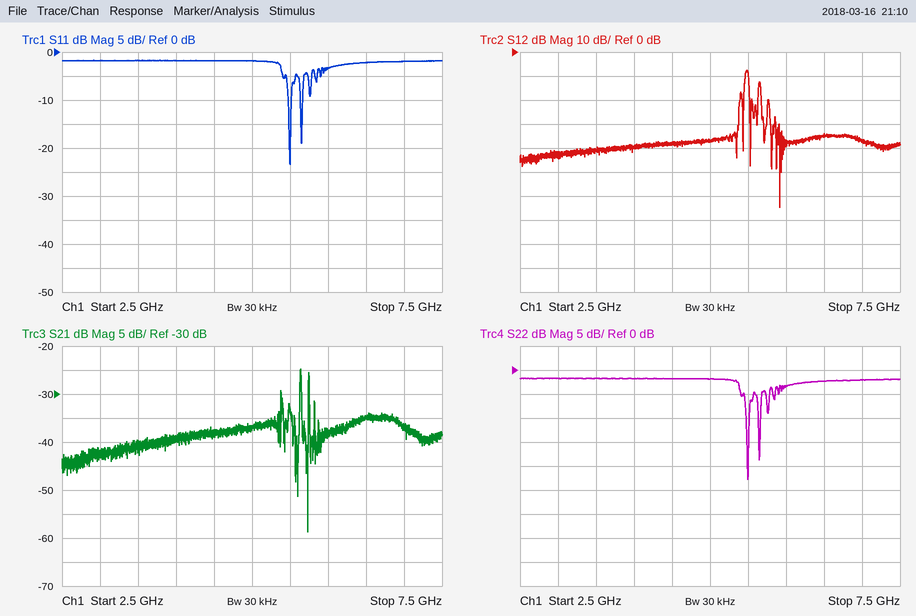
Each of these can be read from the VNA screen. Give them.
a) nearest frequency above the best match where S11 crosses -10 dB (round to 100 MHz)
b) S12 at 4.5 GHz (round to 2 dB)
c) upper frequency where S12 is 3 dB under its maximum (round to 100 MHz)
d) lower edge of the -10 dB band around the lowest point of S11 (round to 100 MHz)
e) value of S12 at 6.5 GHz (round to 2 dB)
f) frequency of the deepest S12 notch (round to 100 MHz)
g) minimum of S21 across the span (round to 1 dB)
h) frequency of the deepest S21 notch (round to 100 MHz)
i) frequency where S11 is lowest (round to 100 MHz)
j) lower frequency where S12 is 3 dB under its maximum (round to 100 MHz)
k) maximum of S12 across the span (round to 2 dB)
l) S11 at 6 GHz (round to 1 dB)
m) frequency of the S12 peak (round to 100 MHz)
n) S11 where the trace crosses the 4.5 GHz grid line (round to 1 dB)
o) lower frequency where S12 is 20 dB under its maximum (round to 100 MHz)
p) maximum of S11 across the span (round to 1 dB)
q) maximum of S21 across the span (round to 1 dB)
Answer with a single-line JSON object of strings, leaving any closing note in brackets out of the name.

{"nearest frequency above the best match where S11 crosses -10 dB": "5.5 GHz", "S12 at 4.5 GHz": "-38 dB", "upper frequency where S12 is 3 dB under its maximum": "5.5 GHz", "lower edge of the -10 dB band around the lowest point of S11": "5.5 GHz", "value of S12 at 6.5 GHz": "-34 dB", "frequency of the deepest S12 notch": "5.9 GHz", "minimum of S21 across the span": "-59 dB", "frequency of the deepest S21 notch": "5.7 GHz", "frequency where S11 is lowest": "5.5 GHz", "lower frequency where S12 is 3 dB under its maximum": "5.5 GHz", "maximum of S12 across the span": "-8 dB", "S11 at 6 GHz": "-3 dB", "frequency of the S12 peak": "5.5 GHz", "S11 where the trace crosses the 4.5 GHz grid line": "-2 dB", "lower frequency where S12 is 20 dB under its maximum": "5.4 GHz", "maximum of S11 across the span": "-2 dB", "maximum of S21 across the span": "-25 dB"}
